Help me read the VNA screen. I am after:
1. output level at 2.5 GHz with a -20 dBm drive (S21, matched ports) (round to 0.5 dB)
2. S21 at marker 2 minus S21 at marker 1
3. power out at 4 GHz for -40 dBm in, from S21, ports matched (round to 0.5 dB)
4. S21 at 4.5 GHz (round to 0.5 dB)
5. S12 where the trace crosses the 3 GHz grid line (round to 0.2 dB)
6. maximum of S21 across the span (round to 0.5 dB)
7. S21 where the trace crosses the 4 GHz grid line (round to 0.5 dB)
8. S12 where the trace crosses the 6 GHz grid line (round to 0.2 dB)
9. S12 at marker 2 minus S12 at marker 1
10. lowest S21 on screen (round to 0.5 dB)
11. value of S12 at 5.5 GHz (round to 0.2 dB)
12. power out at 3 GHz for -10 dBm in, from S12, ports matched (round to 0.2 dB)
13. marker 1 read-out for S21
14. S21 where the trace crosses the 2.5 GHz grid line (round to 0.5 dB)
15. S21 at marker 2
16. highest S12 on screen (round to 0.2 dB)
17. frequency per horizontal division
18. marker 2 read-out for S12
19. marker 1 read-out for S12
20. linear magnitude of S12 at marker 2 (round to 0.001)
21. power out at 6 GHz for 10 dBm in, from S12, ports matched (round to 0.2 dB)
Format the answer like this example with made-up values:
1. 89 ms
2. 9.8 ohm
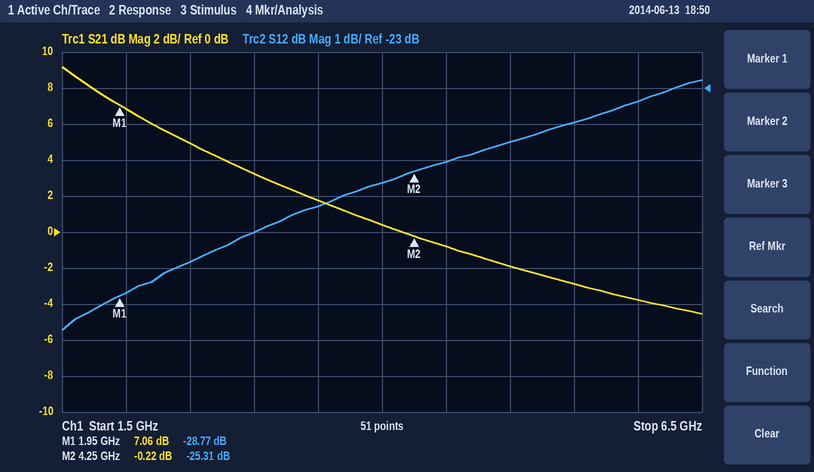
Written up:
1. -15.0 dBm
2. -7.28 dB
3. -39.5 dBm
4. -1.0 dB
5. -27.0 dB
6. 9.0 dB
7. 0.5 dB
8. -23.4 dB
9. 3.46 dB
10. -4.5 dB
11. -24.0 dB
12. -37.0 dBm
13. 7.06 dB
14. 5.0 dB
15. -0.22 dB
16. -22.8 dB
17. 500 MHz
18. -25.31 dB
19. -28.77 dB
20. 0.054
21. -13.4 dBm
